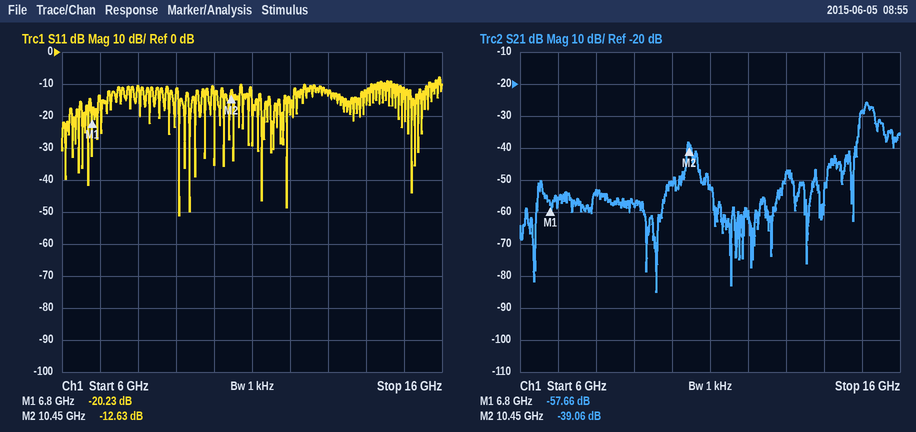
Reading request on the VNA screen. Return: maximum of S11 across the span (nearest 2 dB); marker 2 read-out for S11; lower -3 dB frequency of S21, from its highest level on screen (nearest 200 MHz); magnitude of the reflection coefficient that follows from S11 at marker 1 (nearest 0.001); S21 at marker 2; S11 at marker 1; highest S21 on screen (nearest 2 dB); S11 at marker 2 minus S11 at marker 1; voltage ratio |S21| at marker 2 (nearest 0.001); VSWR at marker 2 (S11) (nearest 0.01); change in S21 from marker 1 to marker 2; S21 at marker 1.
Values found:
-8 dB
-12.63 dB
15.0 GHz
0.097
-39.06 dB
-20.23 dB
-26 dB
7.60 dB
0.011
1.61
18.60 dB
-57.66 dB
